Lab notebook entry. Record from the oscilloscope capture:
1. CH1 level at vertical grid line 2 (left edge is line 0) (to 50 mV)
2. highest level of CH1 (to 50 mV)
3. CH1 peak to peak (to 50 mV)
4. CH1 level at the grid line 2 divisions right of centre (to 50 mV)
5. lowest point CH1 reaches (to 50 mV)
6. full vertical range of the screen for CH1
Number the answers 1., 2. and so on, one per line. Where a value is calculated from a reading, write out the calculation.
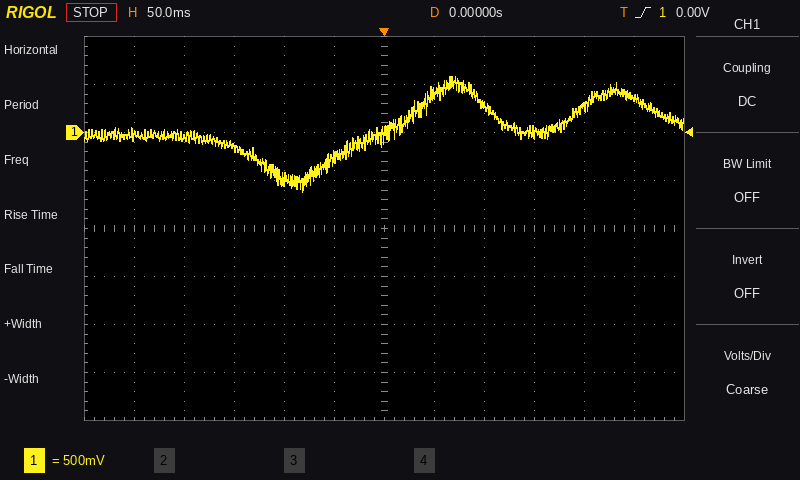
1. -50 mV
2. 600 mV
3. 600 mV − (-600 mV) = 1.20 V
4. 300 mV
5. -600 mV
6. 4 V
